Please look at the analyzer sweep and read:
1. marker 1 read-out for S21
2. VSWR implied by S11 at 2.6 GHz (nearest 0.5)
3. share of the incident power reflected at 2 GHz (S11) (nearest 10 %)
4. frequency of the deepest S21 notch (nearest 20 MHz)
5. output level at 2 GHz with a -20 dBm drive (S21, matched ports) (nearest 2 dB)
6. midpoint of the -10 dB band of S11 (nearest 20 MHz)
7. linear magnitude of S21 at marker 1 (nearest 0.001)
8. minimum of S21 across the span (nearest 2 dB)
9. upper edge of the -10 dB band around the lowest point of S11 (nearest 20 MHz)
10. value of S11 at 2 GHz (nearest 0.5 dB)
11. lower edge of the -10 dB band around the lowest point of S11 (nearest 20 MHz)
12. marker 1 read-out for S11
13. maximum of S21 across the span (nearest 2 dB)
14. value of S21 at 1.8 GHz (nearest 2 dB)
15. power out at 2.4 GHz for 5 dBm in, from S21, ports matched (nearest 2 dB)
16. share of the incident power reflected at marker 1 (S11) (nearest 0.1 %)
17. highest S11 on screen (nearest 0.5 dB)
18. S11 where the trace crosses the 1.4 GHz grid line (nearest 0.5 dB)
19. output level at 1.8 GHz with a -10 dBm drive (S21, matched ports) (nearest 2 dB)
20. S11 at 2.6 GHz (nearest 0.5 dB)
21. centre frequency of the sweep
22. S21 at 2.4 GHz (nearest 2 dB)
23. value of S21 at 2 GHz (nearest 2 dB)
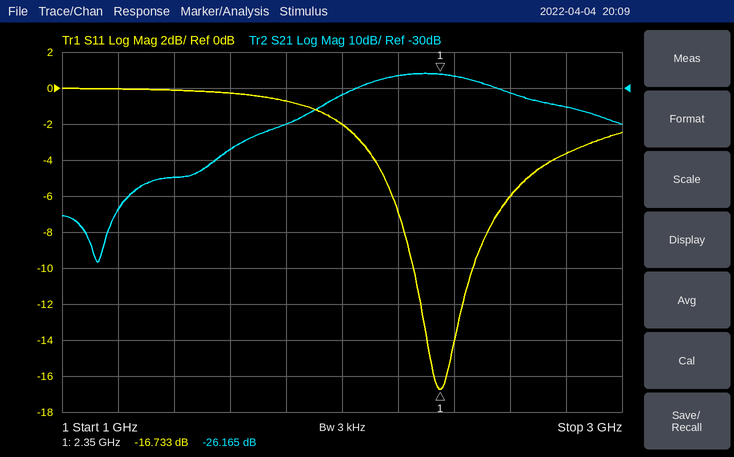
-26.165 dB
3.0
60 %
1.12 GHz
-52 dBm
2.36 GHz
0.049
-78 dB
2.46 GHz
-2.0 dB
2.26 GHz
-16.733 dB
-26 dB
-40 dB
-22 dBm
2.1 %
0.0 dB
0.0 dB
-50 dBm
-6.0 dB
2 GHz
-26 dB
-32 dB
